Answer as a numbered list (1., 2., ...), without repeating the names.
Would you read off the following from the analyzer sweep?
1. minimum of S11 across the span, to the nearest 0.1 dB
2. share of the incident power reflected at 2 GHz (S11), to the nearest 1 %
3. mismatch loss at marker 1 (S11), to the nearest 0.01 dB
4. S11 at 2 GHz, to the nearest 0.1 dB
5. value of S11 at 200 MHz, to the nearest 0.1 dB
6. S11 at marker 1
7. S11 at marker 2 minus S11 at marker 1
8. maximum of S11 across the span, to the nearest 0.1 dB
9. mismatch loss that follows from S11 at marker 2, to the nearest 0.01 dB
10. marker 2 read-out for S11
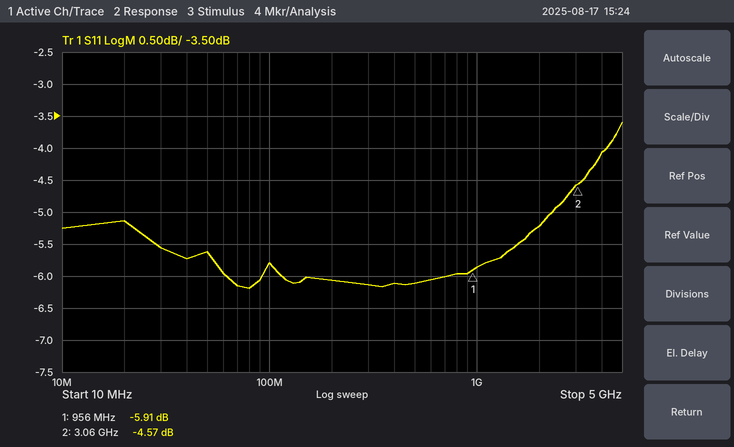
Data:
1. -6.2 dB
2. 30 %
3. 1.29 dB
4. -5.2 dB
5. -6.1 dB
6. -5.91 dB
7. 1.34 dB
8. -3.6 dB
9. 1.87 dB
10. -4.57 dB
